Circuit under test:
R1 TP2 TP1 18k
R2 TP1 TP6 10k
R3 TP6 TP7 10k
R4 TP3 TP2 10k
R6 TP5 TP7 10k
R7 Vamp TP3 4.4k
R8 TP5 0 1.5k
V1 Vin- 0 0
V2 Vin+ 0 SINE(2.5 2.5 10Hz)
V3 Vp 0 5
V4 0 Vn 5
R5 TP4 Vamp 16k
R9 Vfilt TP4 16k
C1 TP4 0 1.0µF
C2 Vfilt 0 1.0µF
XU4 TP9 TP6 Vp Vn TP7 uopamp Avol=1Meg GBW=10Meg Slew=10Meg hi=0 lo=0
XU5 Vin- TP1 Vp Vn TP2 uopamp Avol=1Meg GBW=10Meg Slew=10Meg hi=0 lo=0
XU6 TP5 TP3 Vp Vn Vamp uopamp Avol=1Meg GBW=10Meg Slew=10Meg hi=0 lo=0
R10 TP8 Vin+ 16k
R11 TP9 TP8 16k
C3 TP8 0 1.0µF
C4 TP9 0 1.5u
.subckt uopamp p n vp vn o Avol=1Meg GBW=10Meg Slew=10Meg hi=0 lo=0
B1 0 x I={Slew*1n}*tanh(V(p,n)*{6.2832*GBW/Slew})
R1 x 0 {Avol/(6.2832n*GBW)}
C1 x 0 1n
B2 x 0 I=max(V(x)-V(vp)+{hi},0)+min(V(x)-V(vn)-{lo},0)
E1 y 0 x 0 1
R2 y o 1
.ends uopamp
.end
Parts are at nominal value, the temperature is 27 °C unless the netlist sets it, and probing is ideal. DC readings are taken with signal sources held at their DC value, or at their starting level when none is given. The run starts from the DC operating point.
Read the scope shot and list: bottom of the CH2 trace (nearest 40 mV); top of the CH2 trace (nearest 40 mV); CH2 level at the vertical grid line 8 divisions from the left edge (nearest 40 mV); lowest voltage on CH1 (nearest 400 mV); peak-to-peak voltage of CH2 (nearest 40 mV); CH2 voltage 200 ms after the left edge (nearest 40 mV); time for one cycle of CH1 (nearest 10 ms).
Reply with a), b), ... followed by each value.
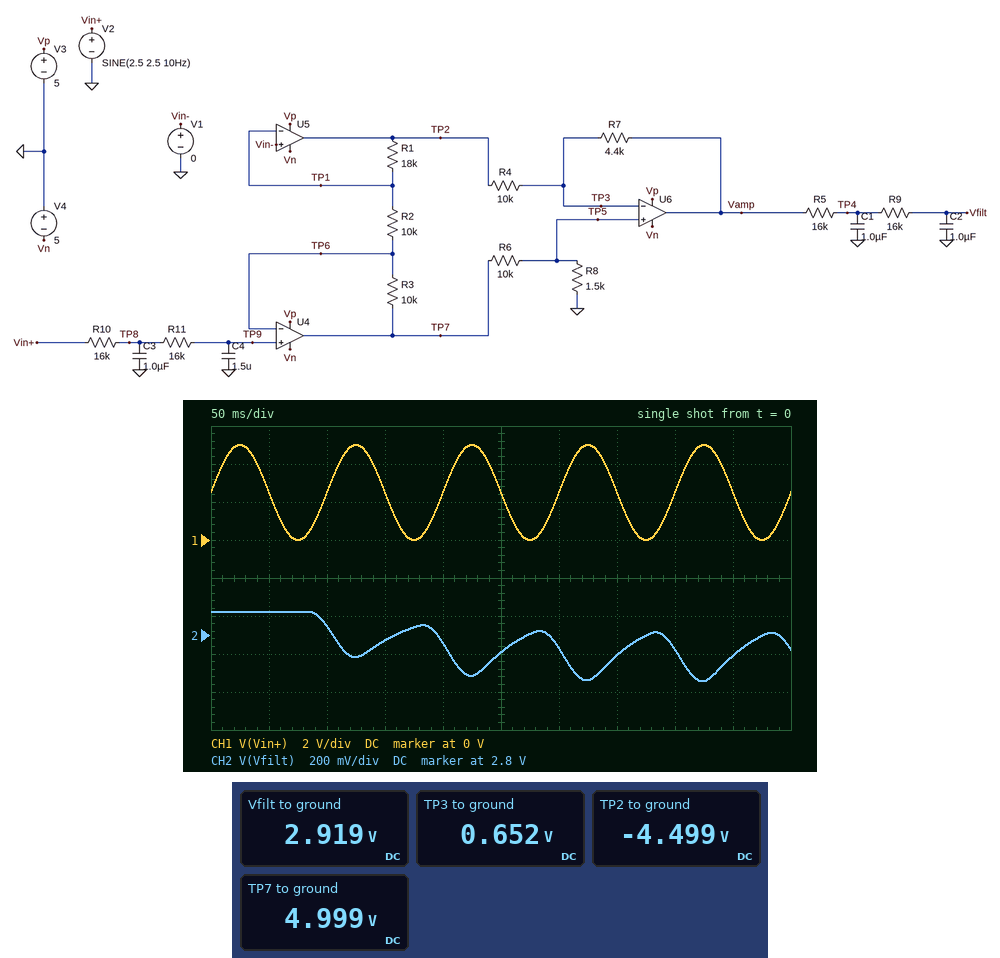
a) 2.56 V
b) 2.92 V
c) 2.72 V
d) 0 V
e) 360 mV
f) 2.76 V
g) 100 ms
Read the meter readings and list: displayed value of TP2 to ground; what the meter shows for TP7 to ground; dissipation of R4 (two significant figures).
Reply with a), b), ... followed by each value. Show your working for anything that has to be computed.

a) -4.499 V
b) 4.999 V
c) (652 mV - (-4.499 V))^2 / 10 kΩ = 2.7 mW
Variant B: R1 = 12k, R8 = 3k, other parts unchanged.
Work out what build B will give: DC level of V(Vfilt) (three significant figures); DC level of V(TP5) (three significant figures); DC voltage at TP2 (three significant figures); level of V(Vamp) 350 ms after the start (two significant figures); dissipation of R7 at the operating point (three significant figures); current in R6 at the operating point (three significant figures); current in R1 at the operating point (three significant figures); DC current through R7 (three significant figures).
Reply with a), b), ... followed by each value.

a) 2.98 V
b) 1.15 V
c) -3.00 V
d) 3.0 V
e) 759 µW
f) 385 µA
g) 250 µA
h) 415 µA
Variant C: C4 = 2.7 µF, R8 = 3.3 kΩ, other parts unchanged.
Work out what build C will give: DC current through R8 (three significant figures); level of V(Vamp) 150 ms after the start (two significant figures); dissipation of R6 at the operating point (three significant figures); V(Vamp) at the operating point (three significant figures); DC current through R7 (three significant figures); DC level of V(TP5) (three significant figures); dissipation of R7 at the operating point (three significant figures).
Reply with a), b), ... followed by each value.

a) 376 µA
b) 3.8 V
c) 1.41 mW
d) 3.77 V
e) 574 µA
f) 1.24 V
g) 1.45 mW
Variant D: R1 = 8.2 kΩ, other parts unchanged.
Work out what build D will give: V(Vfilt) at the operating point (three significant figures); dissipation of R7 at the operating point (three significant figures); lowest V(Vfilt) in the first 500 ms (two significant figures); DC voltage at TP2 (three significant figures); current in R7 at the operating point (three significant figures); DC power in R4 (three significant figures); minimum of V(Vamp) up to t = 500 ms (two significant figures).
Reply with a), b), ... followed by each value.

a) 1.84 V
b) 321 µW
c) 1.6 V
d) -2.05 V
e) 270 µA
f) 730 µW
g) 1.4 V
